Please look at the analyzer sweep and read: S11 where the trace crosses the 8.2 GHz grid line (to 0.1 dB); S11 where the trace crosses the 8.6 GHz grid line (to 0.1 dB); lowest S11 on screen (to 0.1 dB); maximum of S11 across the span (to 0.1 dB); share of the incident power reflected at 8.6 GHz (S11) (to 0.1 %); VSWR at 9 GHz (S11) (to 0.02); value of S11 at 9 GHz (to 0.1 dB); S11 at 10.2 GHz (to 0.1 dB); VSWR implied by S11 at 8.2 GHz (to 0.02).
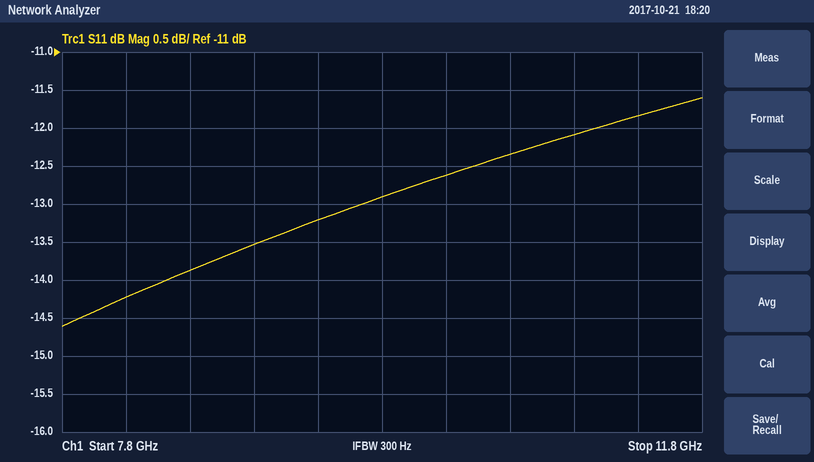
-14.2 dB
-13.9 dB
-14.6 dB
-11.6 dB
4.1 %
1.54
-13.5 dB
-12.6 dB
1.48
